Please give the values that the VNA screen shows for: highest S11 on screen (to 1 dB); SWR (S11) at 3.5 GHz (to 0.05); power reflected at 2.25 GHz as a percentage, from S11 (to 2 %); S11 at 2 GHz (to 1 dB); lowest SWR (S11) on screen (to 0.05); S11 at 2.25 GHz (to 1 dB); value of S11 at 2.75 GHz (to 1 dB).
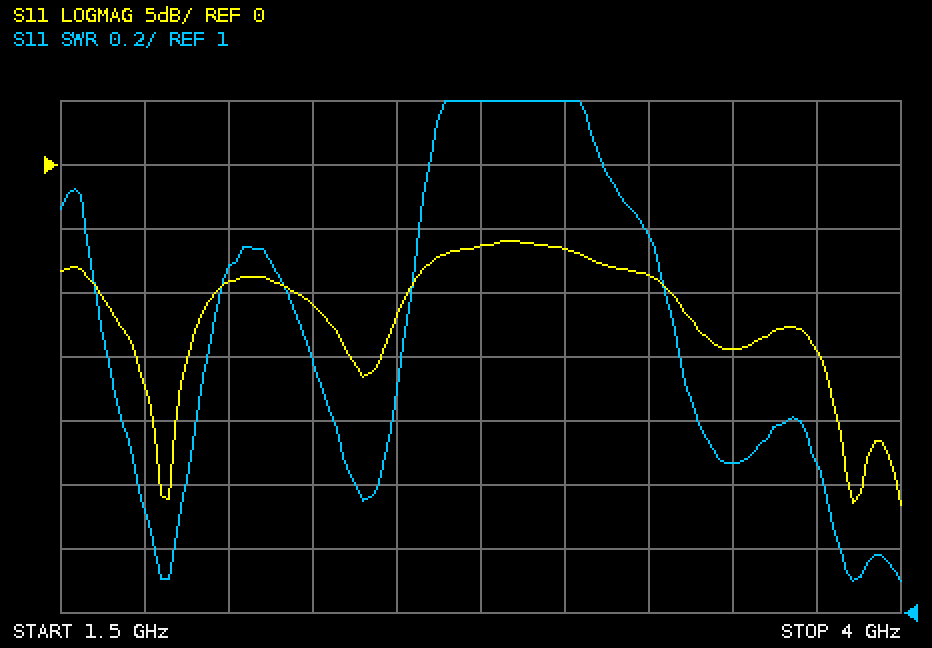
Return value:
-6 dB
1.45
8 %
-9 dB
1.10
-11 dB
-6 dB
